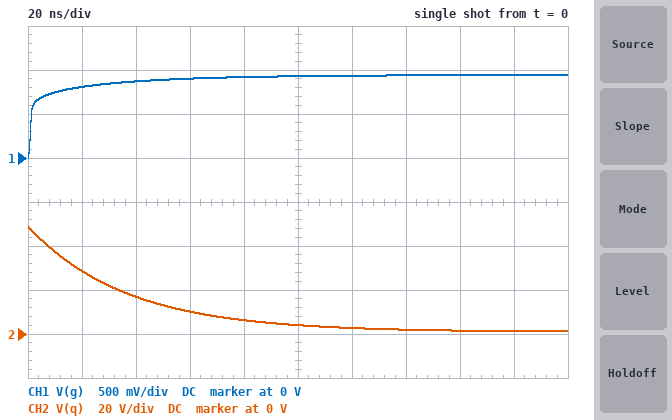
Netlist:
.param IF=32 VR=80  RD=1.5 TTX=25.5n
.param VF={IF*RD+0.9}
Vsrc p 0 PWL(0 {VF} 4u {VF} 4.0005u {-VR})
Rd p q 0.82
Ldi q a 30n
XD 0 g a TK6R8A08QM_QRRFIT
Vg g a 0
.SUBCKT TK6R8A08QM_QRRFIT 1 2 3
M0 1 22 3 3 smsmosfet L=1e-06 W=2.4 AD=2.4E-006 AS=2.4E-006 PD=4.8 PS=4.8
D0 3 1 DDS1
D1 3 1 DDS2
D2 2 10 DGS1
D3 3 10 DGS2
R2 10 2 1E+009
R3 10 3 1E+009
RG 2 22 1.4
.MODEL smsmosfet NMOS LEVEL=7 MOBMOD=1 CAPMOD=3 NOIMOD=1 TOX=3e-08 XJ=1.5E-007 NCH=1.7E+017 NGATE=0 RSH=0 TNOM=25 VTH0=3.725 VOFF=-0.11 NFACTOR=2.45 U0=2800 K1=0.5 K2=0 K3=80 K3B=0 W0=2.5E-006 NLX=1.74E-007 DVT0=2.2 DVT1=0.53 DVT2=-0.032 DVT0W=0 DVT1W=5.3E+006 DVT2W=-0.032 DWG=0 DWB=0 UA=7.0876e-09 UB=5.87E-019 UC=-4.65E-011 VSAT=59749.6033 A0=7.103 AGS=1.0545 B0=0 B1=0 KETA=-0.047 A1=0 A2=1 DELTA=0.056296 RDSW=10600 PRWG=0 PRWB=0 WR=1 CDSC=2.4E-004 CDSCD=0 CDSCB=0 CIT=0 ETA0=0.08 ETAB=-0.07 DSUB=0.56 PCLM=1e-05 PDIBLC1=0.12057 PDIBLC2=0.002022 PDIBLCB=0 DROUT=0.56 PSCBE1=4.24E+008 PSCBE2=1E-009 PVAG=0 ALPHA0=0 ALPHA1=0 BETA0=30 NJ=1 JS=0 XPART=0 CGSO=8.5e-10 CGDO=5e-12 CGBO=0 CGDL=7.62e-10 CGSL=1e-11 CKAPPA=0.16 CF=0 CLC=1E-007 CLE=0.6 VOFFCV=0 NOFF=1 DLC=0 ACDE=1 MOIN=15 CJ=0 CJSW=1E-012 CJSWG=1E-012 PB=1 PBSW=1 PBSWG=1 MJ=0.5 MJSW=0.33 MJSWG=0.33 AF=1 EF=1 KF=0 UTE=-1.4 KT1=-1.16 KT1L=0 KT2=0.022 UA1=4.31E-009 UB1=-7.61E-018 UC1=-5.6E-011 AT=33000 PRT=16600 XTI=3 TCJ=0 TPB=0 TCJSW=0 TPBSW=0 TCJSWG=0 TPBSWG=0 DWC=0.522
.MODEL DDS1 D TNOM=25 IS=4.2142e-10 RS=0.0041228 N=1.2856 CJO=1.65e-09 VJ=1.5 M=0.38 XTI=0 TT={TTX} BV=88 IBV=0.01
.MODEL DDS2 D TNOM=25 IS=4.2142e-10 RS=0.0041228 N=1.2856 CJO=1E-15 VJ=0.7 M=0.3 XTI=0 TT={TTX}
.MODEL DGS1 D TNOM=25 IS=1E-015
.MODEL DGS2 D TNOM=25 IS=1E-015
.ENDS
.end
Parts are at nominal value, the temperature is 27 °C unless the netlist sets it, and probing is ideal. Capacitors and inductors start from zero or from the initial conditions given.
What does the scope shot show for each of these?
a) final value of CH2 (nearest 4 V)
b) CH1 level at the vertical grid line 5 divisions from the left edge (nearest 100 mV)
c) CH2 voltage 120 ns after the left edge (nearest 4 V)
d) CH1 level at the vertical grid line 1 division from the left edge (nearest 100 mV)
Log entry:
0 V
900 mV
4 V
800 mV
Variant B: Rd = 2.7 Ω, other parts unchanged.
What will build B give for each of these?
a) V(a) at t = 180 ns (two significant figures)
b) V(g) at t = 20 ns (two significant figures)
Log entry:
820 mV
780 mV
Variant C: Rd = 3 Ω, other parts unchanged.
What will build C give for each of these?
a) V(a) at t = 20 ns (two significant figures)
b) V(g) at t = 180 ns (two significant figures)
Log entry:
770 mV
810 mV
